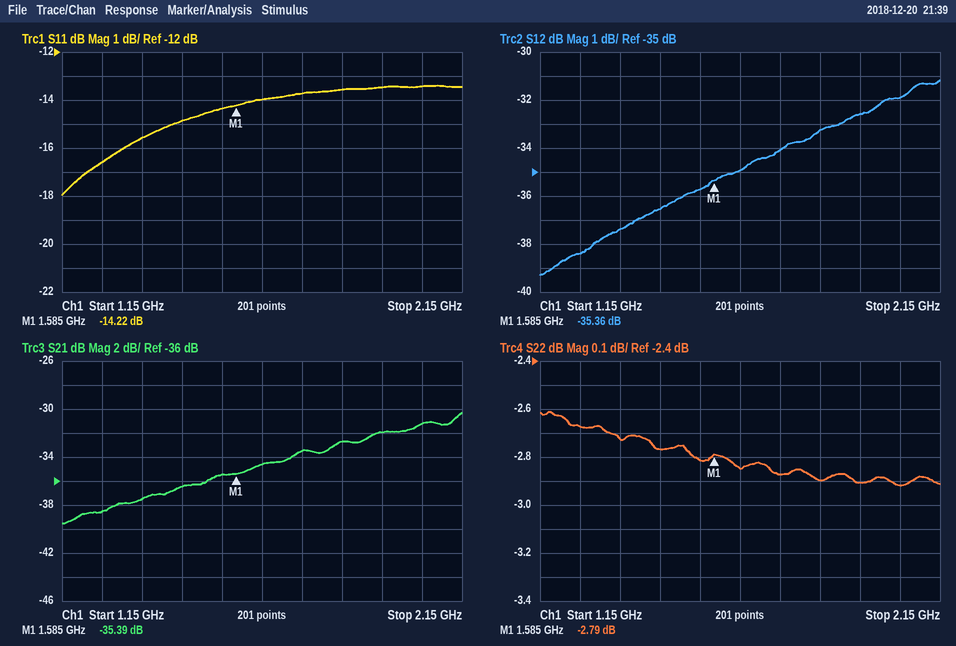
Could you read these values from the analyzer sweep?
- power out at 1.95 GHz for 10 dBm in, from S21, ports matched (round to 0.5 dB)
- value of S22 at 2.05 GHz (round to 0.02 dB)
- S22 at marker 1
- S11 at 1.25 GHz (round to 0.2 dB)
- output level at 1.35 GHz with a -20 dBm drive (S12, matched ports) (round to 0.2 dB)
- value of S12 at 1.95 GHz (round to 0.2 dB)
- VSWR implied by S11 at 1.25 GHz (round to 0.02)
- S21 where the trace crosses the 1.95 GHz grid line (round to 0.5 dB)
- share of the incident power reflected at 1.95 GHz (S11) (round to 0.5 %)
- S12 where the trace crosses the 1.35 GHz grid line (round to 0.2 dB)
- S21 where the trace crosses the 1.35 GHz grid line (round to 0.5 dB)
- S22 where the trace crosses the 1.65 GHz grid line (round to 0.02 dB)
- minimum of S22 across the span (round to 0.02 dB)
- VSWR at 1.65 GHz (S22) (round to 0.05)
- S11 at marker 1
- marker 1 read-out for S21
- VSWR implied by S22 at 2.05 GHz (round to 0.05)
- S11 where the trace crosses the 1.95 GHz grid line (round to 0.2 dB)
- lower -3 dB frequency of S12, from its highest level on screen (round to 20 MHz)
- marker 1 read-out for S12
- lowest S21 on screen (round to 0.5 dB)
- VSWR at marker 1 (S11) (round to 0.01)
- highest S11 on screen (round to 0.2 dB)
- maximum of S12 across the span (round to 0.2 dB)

-22.0 dBm
-2.92 dB
-2.79 dB
-16.6 dB
-57.4 dBm
-32.6 dB
1.34
-32.0 dB
4.5 %
-37.4 dB
-37.5 dB
-2.84 dB
-2.92 dB
6.15
-14.22 dB
-35.39 dB
6.00
-13.4 dB
1.74 GHz
-35.36 dB
-39.5 dB
1.48
-13.4 dB
-31.2 dB
